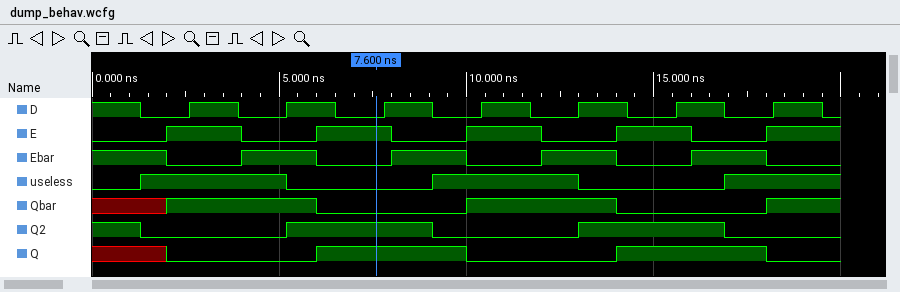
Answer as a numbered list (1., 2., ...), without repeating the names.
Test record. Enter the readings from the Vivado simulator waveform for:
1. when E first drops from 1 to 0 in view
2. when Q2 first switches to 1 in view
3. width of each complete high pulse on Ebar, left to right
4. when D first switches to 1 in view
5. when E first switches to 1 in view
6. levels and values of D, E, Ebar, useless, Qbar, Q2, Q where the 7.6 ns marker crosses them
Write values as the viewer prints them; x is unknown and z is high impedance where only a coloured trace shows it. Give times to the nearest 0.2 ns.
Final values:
1. 4 ns
2. 5.2 ns
3. 2 ns, 2 ns, 2 ns, 2 ns
4. 2.6 ns
5. 2 ns
6. D=0, E=1, Ebar=0, useless=0, Qbar=0, Q2=1, Q=1
